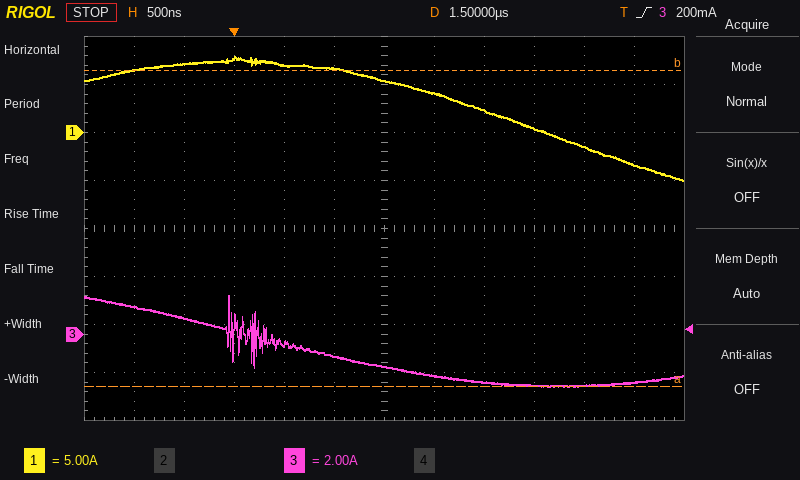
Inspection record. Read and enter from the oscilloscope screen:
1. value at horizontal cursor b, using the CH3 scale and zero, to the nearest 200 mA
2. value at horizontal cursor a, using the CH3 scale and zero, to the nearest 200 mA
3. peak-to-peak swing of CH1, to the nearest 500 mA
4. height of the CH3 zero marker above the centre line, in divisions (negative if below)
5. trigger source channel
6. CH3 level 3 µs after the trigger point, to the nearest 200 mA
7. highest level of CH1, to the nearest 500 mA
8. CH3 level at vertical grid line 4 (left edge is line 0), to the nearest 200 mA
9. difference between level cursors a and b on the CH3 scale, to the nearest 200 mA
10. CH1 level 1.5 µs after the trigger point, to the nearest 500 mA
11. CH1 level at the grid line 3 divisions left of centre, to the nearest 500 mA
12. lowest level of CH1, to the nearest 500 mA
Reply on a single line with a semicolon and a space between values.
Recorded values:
11.0 A; -2.2 A; 13.0 A; -2.2 div; CH3; -2.2 A; 8.0 A; -400 mA; 13.2 A; 5.5 A; 7.5 A; -5.0 A
